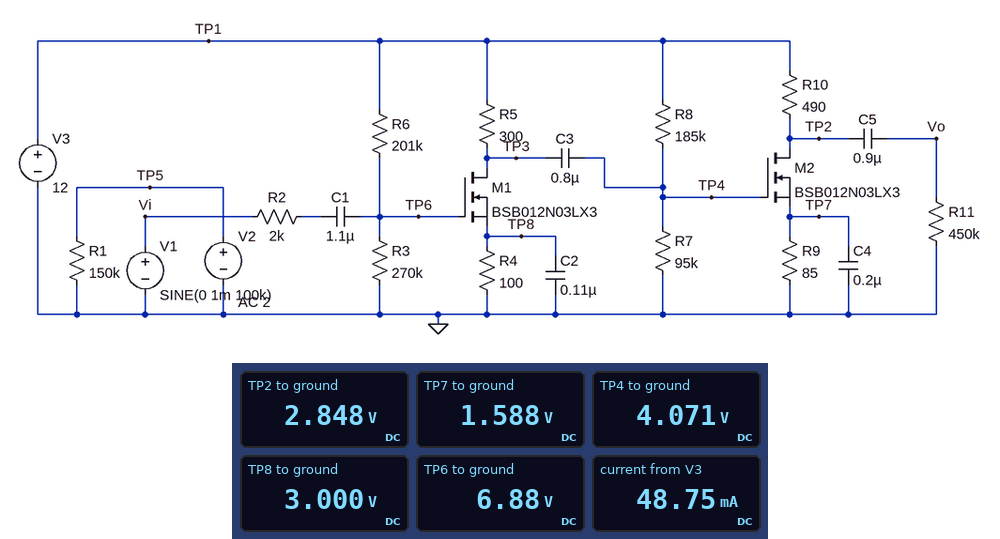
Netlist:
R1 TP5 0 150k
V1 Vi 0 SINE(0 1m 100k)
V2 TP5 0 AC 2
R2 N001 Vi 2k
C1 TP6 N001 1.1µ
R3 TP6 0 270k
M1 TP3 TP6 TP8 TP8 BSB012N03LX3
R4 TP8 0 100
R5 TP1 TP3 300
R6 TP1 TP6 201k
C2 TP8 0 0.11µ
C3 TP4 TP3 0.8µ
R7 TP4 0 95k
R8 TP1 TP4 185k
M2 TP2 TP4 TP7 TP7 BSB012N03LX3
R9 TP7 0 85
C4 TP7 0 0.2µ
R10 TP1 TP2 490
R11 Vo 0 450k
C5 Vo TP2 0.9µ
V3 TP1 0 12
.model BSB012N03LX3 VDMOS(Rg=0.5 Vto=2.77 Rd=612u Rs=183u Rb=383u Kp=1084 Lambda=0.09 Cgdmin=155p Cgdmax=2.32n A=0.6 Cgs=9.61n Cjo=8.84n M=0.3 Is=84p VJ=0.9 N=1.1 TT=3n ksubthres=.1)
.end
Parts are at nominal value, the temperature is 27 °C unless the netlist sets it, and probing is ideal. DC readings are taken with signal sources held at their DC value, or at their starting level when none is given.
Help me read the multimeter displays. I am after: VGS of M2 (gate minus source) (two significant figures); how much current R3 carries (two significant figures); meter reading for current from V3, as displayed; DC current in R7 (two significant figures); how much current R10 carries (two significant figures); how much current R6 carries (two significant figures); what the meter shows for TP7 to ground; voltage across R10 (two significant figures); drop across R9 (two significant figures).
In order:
2.5 V
25 µA
48.75 mA
43 µA
19 mA
25 µA
1.588 V
9.2 V
1.6 V
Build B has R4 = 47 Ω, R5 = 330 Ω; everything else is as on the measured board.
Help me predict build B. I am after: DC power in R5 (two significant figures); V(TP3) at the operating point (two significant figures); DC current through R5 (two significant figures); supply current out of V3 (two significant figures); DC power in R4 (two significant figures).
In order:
330 mW
1.5 V
32 mA
51 mA
48 mW
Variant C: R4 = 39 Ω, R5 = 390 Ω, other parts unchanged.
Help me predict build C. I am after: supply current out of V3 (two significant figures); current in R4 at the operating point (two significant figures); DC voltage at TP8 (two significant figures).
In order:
47 mA
28 mA
1.1 V
